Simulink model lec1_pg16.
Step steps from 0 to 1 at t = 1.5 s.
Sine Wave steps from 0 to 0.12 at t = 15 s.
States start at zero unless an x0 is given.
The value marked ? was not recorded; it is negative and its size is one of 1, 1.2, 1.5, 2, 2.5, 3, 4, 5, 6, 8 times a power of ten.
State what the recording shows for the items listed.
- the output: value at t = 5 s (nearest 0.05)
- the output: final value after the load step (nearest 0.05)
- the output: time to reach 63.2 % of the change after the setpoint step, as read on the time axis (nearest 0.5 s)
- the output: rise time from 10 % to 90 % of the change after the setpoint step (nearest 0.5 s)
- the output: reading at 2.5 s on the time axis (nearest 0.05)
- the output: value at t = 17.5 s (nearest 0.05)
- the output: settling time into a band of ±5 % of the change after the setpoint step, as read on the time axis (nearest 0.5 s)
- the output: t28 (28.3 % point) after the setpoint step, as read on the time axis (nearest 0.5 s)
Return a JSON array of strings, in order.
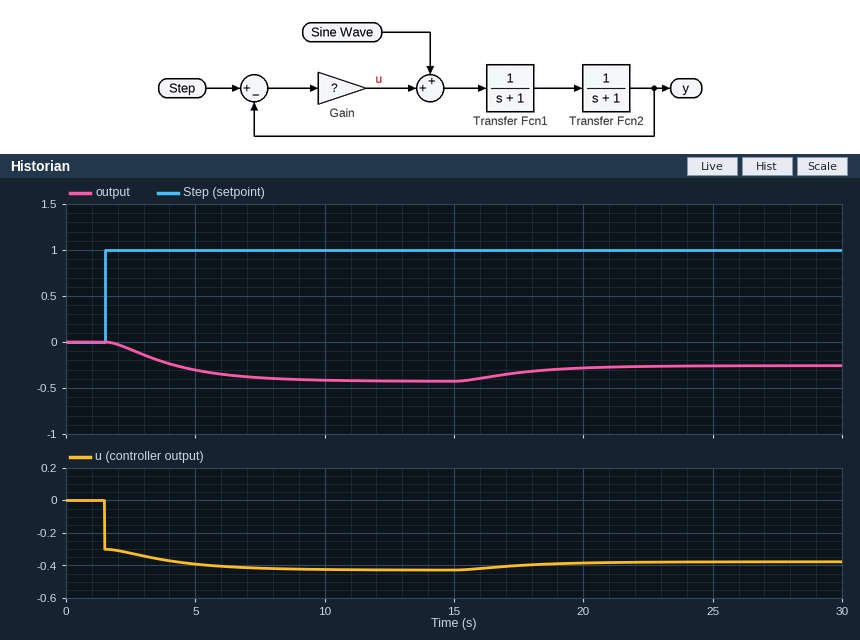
["-0.30", "-0.25", "4.5 s", "5.0 s", "-0.10", "-0.35", "9.0 s", "3.0 s"]
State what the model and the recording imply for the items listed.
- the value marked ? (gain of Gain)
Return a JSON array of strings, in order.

["-0.3"]
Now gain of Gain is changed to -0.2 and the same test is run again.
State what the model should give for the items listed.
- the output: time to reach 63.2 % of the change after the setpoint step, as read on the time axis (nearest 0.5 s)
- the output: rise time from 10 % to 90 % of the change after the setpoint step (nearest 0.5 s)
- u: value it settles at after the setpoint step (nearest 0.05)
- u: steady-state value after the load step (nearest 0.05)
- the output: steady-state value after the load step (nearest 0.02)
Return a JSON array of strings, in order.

["4.0 s", "4.5 s", "-0.25", "-0.20", "-0.10"]
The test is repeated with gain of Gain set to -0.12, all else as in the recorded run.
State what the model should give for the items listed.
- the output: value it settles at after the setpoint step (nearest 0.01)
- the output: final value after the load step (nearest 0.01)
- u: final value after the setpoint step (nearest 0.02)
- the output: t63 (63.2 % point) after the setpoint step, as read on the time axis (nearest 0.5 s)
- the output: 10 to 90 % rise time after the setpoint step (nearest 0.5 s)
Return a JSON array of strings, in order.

["-0.14", "0.00", "-0.14", "4.0 s", "4.0 s"]
